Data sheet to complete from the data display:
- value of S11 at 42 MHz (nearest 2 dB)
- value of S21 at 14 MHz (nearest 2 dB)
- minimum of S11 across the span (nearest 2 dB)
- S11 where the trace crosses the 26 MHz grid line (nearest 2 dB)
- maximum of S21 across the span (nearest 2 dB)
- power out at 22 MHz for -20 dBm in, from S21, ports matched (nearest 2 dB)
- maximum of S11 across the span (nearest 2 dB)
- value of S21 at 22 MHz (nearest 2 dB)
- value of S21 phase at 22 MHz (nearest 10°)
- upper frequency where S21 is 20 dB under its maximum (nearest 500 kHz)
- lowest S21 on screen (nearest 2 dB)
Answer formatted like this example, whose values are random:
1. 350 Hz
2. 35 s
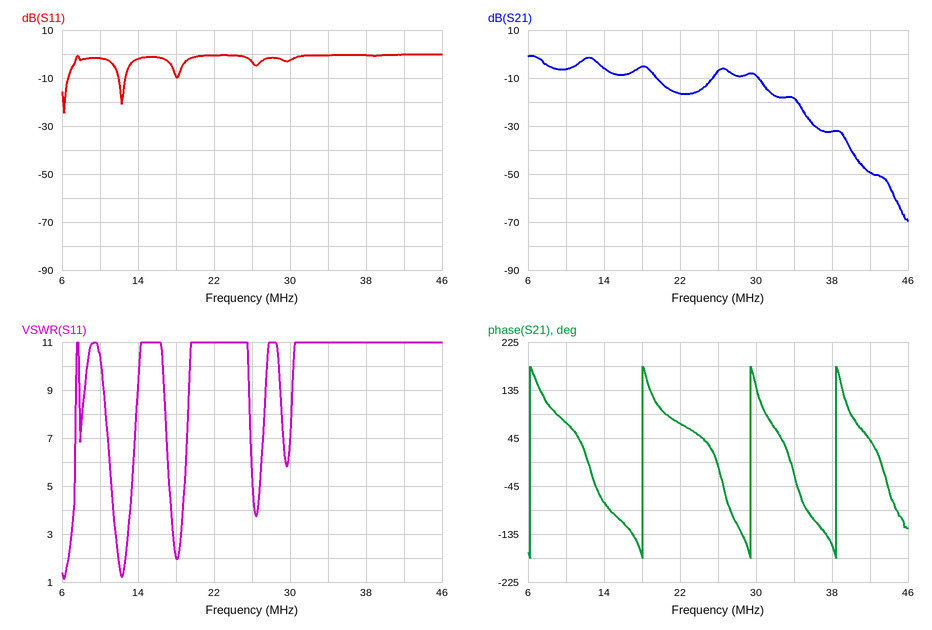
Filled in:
1. 0 dB
2. -6 dB
3. -24 dB
4. -4 dB
5. 0 dB
6. -36 dBm
7. 0 dB
8. -16 dB
9. 70°
10. 34.5 MHz
11. -70 dB
